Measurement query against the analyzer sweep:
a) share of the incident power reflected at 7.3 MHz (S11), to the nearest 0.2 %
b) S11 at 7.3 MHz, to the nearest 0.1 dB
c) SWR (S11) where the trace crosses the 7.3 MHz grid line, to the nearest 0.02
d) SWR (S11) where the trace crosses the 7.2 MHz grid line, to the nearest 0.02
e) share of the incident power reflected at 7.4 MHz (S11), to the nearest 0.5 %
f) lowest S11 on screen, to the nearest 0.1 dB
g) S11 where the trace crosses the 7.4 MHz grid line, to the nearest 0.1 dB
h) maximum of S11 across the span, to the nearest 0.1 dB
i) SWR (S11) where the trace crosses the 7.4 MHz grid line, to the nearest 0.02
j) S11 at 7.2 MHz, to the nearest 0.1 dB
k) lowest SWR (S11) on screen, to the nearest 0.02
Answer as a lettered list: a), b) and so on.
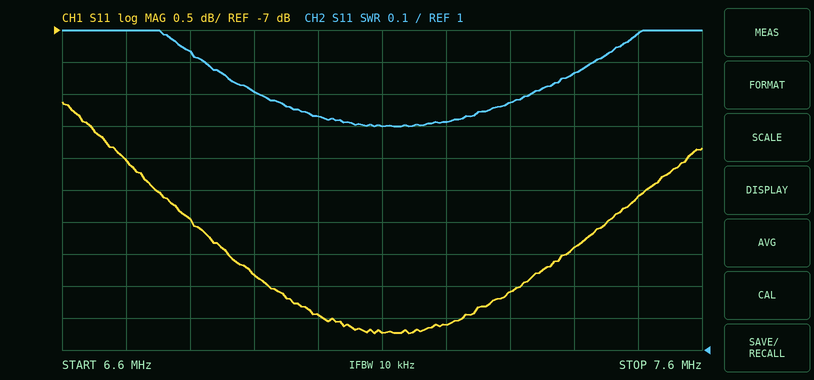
a) 7.8 %
b) -11.1 dB
c) 1.78
d) 1.72
e) 9.0 %
f) -11.7 dB
g) -10.4 dB
h) -8.1 dB
i) 1.86
j) -11.6 dB
k) 1.70
